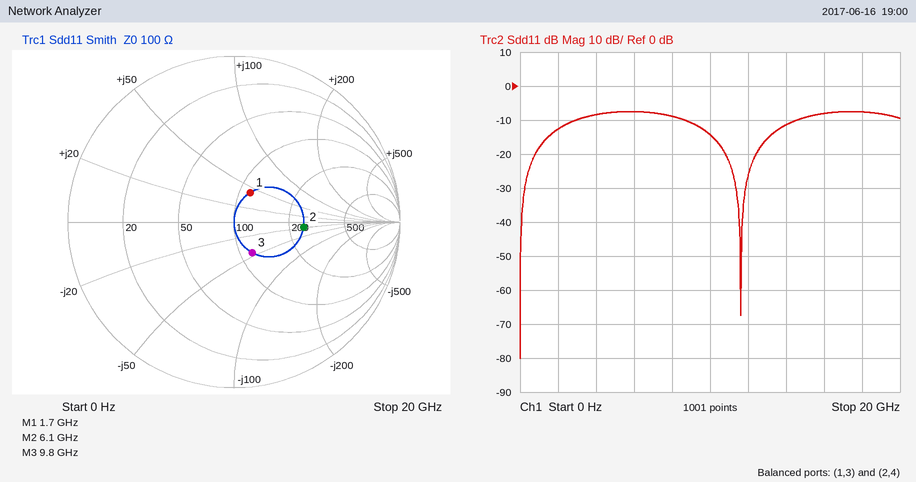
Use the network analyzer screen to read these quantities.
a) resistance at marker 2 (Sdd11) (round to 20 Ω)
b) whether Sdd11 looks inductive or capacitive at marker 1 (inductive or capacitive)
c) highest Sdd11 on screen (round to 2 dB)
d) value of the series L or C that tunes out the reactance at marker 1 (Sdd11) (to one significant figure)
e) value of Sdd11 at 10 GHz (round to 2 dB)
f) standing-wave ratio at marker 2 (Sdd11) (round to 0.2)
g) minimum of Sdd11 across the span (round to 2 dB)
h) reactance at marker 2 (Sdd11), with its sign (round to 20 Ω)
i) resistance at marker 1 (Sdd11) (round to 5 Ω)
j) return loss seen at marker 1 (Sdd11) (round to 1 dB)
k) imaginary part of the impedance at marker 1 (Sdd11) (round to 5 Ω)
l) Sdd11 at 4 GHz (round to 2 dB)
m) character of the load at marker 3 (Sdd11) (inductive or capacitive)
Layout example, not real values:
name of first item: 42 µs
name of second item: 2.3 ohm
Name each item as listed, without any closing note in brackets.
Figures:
resistance at marker 2 (Sdd11): 240 Ω
whether Sdd11 looks inductive or capacitive at marker 1: inductive
highest Sdd11 on screen: -8 dB
value of the series L or C that tunes out the reactance at marker 1 (Sdd11): 2 pF
value of Sdd11 at 10 GHz: -14 dB
standing-wave ratio at marker 2 (Sdd11): 2.4
minimum of Sdd11 across the span: -80 dB
reactance at marker 2 (Sdd11), with its sign: -20 Ω
resistance at marker 1 (Sdd11): 115 Ω
return loss seen at marker 1 (Sdd11): 14 dB
imaginary part of the impedance at marker 1 (Sdd11): +40 Ω
Sdd11 at 4 GHz: -8 dB
character of the load at marker 3 (Sdd11): capacitive
